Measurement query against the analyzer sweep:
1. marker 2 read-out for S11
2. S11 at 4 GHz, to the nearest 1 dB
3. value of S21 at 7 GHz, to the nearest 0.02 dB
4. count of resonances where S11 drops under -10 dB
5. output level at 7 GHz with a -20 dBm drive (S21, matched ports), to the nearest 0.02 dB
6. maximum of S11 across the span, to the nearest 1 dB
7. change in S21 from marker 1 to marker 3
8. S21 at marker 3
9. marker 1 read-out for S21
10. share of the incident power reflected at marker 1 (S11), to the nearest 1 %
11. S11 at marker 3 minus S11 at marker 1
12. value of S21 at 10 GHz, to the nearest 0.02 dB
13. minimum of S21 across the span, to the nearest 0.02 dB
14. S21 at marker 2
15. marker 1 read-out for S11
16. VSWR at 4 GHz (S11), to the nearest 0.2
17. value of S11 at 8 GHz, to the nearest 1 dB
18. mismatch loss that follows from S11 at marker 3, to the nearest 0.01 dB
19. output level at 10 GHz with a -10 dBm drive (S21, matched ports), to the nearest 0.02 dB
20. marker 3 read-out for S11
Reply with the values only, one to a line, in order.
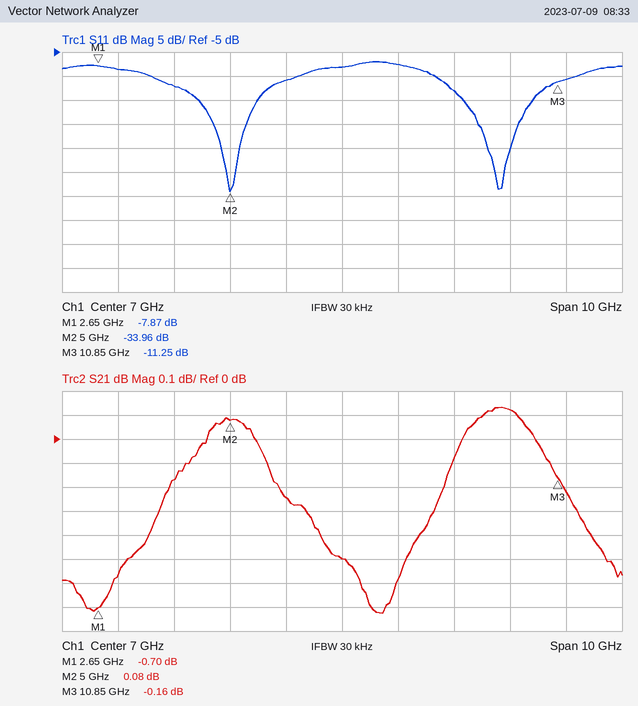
-33.96 dB
-12 dB
-0.50 dB
2
-20.50 dBm
-7 dB
0.54 dB
-0.16 dB
-0.70 dB
16 %
-3.38 dB
0.12 dB
-0.72 dB
0.08 dB
-7.87 dB
1.6
-8 dB
0.34 dB
-9.88 dBm
-11.25 dB
